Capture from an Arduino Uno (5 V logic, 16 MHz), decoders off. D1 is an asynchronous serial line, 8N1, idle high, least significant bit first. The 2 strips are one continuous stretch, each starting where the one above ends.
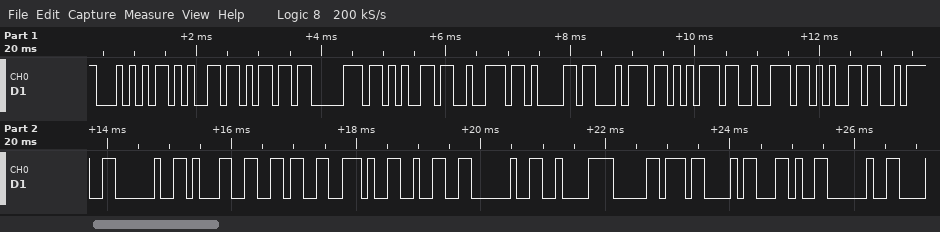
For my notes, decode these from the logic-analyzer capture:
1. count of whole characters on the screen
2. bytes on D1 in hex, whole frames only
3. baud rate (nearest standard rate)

23
0x54 0x65 0x6D 0x70 0x65 0x72 0x61 0x74 0x75 0x72 0x65 0x3A 0x20 0x31 0x36 0x2E 0x32 0x20 0xC2 0xB0 0x43 0x2C 0x20
9600 baud
